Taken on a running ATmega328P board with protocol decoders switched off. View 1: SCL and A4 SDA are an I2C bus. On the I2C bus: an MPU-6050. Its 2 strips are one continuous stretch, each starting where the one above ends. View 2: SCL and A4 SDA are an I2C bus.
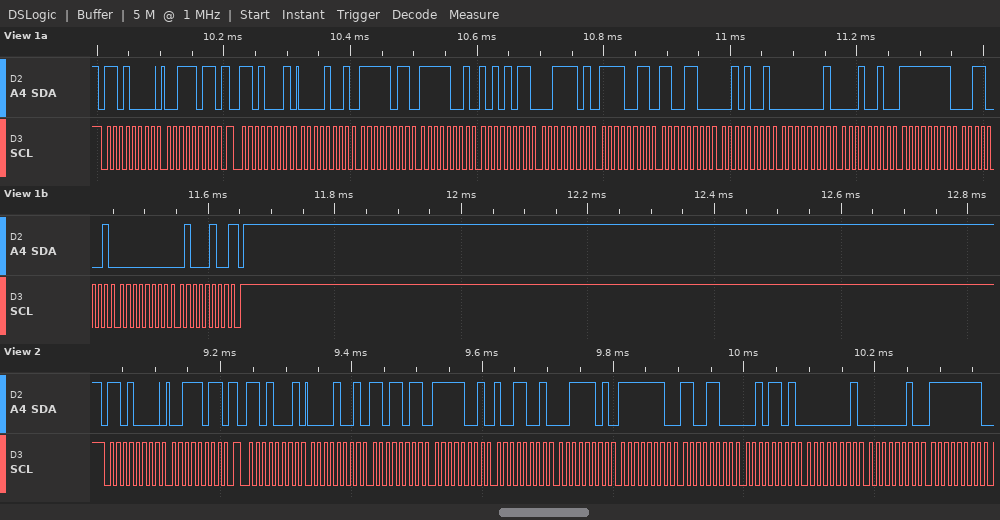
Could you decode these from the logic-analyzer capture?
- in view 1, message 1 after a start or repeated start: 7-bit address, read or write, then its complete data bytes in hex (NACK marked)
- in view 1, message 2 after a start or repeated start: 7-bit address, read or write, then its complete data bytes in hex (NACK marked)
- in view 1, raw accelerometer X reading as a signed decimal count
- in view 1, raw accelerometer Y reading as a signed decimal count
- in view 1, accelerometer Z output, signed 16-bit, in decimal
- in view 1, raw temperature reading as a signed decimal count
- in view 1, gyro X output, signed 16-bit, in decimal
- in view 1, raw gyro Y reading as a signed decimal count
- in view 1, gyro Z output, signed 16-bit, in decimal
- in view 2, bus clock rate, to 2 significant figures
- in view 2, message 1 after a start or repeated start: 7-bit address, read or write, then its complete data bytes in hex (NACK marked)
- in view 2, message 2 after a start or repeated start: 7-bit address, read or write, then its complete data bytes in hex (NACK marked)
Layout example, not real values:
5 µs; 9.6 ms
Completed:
0x68 write: 3B; 0x68 read: 09 FB F9 AB 3D F3 CC 29 01 12 FF 31 00 44 NACK; 2555; -1621; 15859; -13271; 274; -207; 68; 100 kHz; 0x68 write: 3B; 0x68 read: 09 DB F9 99 3D FE CC 2D 01 02 FF
